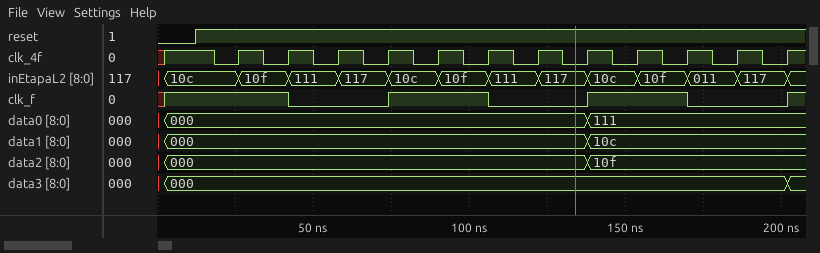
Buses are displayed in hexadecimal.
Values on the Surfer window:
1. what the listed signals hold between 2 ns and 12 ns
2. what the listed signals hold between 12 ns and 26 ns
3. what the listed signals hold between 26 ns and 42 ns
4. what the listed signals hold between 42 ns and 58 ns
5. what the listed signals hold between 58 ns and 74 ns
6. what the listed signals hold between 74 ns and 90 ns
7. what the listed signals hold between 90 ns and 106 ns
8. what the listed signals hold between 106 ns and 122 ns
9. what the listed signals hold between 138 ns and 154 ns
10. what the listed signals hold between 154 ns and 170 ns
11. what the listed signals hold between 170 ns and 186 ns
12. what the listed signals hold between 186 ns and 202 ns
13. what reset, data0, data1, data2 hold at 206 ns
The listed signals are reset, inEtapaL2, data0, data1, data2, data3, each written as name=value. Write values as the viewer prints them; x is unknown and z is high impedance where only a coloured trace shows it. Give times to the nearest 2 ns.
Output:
reset=0, inEtapaL2=10c, data0=000, data1=000, data2=000, data3=000
reset=1, inEtapaL2=10c, data0=000, data1=000, data2=000, data3=000
reset=1, inEtapaL2=10f, data0=000, data1=000, data2=000, data3=000
reset=1, inEtapaL2=111, data0=000, data1=000, data2=000, data3=000
reset=1, inEtapaL2=117, data0=000, data1=000, data2=000, data3=000
reset=1, inEtapaL2=10c, data0=000, data1=000, data2=000, data3=000
reset=1, inEtapaL2=10f, data0=000, data1=000, data2=000, data3=000
reset=1, inEtapaL2=111, data0=000, data1=000, data2=000, data3=000
reset=1, inEtapaL2=10c, data0=111, data1=10c, data2=10f, data3=000
reset=1, inEtapaL2=10f, data0=111, data1=10c, data2=10f, data3=000
reset=1, inEtapaL2=011, data0=111, data1=10c, data2=10f, data3=000
reset=1, inEtapaL2=117, data0=111, data1=10c, data2=10f, data3=000
reset=1, data0=111, data1=10c, data2=10f
